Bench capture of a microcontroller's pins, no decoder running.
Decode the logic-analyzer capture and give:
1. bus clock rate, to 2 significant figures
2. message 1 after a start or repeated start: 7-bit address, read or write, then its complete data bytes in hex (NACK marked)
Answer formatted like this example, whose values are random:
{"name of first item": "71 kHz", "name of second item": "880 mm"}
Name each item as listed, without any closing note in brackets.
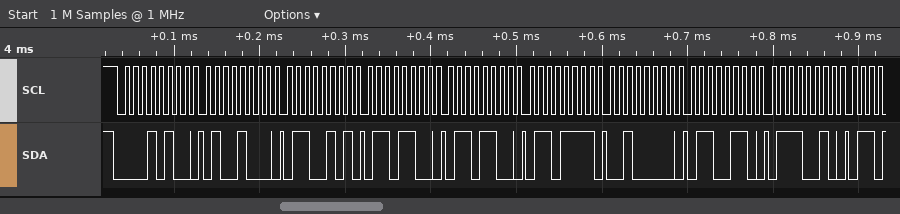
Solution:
{"bus clock rate, to 2 significant figures": "100 kHz", "message 1 after a start or repeated start: 7-bit address, read or write, then its complete data bytes in hex": "0x0A write: 48 65 6C 6C 6F 20 66 72"}
